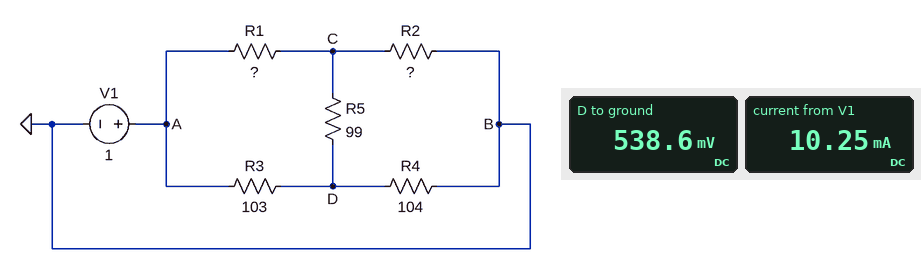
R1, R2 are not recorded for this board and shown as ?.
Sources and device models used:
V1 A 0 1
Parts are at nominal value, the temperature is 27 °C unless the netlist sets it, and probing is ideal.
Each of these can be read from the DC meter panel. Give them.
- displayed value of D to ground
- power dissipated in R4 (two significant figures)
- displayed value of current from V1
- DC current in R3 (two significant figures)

538.6 mV
2.8 mW
10.25 mA
4.5 mA
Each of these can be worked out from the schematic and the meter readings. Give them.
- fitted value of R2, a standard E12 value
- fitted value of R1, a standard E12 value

120 Ω
68 Ω
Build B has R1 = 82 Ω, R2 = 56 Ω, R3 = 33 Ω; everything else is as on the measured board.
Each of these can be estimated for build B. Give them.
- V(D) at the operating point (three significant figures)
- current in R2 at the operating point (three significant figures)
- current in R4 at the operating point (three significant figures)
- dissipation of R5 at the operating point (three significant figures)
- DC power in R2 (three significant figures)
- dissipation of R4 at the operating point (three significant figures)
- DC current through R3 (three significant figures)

703 mV
8.58 mA
6.76 mA
499 µW
4.12 mW
4.75 mW
9.00 mA
